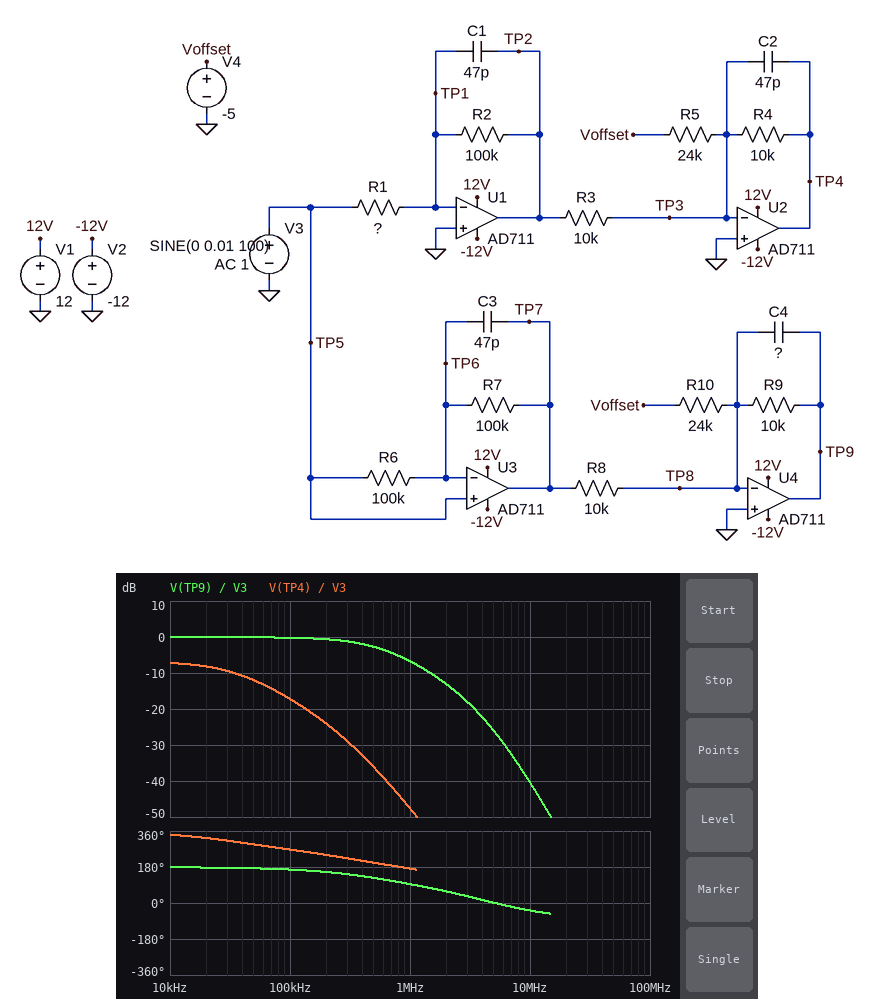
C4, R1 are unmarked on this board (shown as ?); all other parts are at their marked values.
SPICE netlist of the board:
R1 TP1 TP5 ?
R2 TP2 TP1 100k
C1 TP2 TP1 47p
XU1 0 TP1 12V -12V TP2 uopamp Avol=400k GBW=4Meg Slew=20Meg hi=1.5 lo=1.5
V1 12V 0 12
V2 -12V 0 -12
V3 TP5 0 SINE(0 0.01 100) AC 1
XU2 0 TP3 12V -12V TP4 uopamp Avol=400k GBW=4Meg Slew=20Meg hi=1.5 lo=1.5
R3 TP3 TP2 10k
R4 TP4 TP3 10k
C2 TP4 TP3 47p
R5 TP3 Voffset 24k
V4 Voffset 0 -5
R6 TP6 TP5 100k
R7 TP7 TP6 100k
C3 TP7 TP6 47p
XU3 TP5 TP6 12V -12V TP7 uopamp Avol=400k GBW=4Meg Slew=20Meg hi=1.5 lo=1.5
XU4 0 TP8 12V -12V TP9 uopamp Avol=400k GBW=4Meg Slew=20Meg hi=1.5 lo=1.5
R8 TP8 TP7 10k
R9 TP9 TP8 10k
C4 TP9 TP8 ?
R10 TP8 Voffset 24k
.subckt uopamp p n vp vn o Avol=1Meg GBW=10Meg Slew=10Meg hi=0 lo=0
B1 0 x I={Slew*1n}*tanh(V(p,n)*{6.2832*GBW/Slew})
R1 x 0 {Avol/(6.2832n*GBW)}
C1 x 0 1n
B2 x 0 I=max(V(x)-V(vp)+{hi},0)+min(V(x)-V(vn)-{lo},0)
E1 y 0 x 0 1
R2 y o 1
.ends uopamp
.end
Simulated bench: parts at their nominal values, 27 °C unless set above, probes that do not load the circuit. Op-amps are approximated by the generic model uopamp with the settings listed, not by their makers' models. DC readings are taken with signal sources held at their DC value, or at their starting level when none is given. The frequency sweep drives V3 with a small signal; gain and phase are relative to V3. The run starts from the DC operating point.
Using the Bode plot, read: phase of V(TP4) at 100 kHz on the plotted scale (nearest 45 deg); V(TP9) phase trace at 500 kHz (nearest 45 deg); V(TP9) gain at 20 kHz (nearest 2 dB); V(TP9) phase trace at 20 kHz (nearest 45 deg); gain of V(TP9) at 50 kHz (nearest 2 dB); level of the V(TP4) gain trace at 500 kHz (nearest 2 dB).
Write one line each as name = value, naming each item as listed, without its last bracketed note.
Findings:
phase of V(TP4) at 100 kHz on the plotted scale = 270 deg
V(TP9) phase trace at 500 kHz = 135 deg
V(TP9) gain at 20 kHz = 0 dB
V(TP9) phase trace at 20 kHz = 180 deg
gain of V(TP9) at 50 kHz = 0 dB
level of the V(TP4) gain trace at 500 kHz = -36 dB
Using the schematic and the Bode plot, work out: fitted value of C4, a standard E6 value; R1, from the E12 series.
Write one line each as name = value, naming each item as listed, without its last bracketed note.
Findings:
fitted value of C4, a standard E6 value = 22 pF
R1, from the E12 series = 220 kΩ
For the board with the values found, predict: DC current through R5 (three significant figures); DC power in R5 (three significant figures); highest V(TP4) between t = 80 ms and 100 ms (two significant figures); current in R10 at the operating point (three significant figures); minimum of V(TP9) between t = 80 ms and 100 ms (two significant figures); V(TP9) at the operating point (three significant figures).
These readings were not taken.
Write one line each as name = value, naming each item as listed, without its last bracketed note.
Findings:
DC current through R5 = 208 µA
DC power in R5 = 1.04 mW
highest V(TP4) between t = 80 ms and 100 ms = 2.1 V
current in R10 at the operating point = 208 µA
minimum of V(TP9) between t = 80 ms and 100 ms = 2.1 V
V(TP9) at the operating point = 2.08 V
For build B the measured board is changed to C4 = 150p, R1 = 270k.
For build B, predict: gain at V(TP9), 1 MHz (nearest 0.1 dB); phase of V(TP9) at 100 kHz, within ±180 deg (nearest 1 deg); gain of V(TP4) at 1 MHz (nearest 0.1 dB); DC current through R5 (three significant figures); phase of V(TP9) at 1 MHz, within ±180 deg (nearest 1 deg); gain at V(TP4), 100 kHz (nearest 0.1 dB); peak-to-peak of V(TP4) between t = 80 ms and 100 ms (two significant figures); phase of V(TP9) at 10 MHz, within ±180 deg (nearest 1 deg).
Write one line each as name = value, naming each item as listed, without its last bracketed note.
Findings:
gain at V(TP9), 1 MHz = -20.4 dB
phase of V(TP9) at 100 kHz, within ±180 deg = 133 deg
gain of V(TP4) at 1 MHz = -49.4 dB
DC current through R5 = 208 µA
phase of V(TP9) at 1 MHz, within ±180 deg = 68 deg
gain at V(TP4), 100 kHz = -19.0 dB
peak-to-peak of V(TP4) between t = 80 ms and 100 ms = 7.4 mV
phase of V(TP9) at 10 MHz, within ±180 deg = -45 deg
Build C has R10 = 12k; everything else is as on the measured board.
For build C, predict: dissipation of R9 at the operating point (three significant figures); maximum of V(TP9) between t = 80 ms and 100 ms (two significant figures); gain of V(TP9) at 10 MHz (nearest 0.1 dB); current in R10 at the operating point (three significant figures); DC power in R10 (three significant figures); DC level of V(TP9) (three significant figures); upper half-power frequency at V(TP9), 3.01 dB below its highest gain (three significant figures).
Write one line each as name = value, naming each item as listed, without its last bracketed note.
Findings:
dissipation of R9 at the operating point = 1.74 mW
maximum of V(TP9) between t = 80 ms and 100 ms = 4.2 V
gain of V(TP9) at 10 MHz = -40.5 dB
current in R10 at the operating point = 417 µA
DC power in R10 = 2.08 mW
DC level of V(TP9) = 4.17 V
upper half-power frequency at V(TP9), 3.01 dB below its highest gain = 502 kHz
